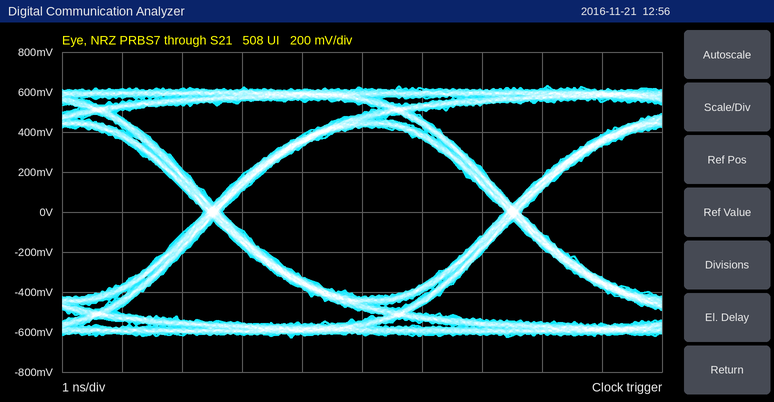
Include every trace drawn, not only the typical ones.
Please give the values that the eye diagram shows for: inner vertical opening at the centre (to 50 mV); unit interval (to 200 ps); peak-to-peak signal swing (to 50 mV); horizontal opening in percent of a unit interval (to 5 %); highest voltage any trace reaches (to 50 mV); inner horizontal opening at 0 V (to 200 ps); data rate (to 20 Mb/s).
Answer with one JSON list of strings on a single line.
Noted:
["850 mV", "5.0 ns", "1.25 V", "95 %", "650 mV", "4.8 ns", "200 Mb/s"]
